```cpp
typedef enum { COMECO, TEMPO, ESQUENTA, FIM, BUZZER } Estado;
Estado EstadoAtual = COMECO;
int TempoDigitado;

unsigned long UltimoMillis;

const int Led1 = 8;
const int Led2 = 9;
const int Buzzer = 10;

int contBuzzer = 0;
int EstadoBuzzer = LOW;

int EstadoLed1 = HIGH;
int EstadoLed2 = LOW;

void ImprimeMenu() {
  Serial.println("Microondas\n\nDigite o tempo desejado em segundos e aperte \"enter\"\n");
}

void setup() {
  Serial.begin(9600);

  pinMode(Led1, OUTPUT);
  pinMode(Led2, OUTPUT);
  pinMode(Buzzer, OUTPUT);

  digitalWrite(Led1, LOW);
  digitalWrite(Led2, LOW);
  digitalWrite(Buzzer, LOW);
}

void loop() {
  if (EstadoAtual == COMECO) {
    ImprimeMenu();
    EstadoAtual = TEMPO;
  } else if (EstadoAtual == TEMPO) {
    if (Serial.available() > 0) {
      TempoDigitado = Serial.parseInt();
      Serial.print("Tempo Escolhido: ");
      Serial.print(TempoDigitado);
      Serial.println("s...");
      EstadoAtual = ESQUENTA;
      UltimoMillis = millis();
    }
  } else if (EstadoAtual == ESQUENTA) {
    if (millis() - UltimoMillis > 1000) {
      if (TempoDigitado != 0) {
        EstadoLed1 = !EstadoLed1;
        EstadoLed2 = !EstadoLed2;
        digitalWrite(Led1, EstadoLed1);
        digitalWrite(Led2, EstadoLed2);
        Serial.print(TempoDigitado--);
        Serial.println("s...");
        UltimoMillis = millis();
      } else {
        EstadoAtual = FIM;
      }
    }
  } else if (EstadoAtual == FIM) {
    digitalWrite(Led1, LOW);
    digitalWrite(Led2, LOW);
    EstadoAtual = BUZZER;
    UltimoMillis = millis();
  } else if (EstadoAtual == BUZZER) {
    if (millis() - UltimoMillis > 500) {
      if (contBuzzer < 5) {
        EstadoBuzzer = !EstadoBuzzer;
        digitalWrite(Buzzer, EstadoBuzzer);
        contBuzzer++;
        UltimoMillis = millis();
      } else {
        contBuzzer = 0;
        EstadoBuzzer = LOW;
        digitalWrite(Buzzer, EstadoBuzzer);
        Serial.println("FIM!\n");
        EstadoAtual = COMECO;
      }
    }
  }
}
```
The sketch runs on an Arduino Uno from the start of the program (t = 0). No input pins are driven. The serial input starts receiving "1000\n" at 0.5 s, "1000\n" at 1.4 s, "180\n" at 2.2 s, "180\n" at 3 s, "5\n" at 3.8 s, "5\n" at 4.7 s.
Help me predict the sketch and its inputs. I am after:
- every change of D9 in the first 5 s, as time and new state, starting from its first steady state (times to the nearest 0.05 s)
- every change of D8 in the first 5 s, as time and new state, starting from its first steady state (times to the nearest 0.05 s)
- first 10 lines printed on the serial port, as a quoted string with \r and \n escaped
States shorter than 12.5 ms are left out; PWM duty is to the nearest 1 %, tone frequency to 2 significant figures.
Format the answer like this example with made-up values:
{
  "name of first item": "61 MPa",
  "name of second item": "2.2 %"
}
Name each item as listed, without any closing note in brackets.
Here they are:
{
  "every change of D9 in the first 5 s, as time and new state, starting from its first steady state": "0 s low; 1.5 s high; 2.5 s low; 3.5 s high; 4.5 s low",
  "every change of D8 in the first 5 s, as time and new state, starting from its first steady state": "0 s low; 2.5 s high; 3.5 s low; 4.5 s high",
  "first 10 lines printed on the serial port, as a quoted string with \\r and \\n escaped": "\"Microondas\\n\\nDigite o tempo desejado em segundos e aperte \\\"enter\\\"\\n\\r\\nTempo Escolhido: 1000s...\\r\\n1000s...\\r\\n999s...\\r\\n998s...\\r\\n997s...\\r\\n996s...\\r\\n\""
}
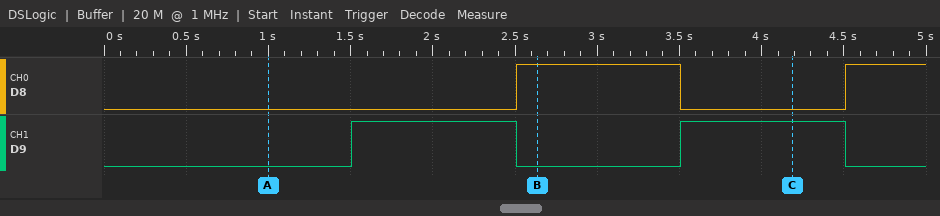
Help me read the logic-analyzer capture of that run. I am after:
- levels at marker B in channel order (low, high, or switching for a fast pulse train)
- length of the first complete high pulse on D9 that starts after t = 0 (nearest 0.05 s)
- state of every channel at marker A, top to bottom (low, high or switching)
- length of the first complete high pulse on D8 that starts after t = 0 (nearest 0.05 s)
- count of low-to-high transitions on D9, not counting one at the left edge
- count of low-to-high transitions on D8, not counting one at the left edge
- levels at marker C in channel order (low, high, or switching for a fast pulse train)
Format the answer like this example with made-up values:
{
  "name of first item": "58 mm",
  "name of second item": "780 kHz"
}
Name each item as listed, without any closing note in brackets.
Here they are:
{
  "levels at marker B in channel order": "D8 high, D9 low",
  "length of the first complete high pulse on D9 that starts after t = 0": "1.00 s",
  "state of every channel at marker A, top to bottom": "D8 low, D9 low",
  "length of the first complete high pulse on D8 that starts after t = 0": "1.00 s",
  "count of low-to-high transitions on D9, not counting one at the left edge": "2",
  "count of low-to-high transitions on D8, not counting one at the left edge": "2",
  "levels at marker C in channel order": "D8 low, D9 high"
}
